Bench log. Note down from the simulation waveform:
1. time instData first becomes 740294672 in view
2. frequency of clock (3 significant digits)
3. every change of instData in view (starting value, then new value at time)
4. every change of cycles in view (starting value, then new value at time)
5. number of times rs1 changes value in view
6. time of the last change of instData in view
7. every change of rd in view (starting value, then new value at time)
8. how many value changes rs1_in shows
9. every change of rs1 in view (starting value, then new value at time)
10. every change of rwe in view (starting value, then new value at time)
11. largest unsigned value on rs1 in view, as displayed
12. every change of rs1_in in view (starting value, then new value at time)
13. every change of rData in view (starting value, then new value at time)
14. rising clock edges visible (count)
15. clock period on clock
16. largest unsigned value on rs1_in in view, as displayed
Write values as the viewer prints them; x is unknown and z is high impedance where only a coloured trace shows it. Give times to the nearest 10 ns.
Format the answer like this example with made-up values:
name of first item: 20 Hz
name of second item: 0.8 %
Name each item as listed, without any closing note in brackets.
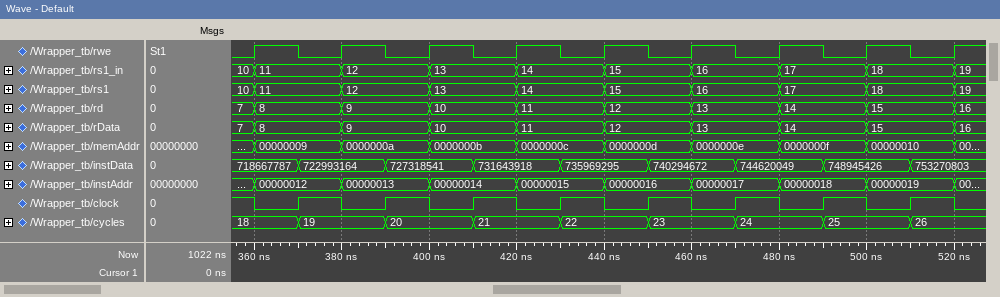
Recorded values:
time instData first becomes 740294672 in view: 450 ns
frequency of clock: 50.0 MHz
every change of instData in view: 718667787, 722993164 at 370 ns, 727318541 at 390 ns, 731643918 at 410 ns, 735969295 at 430 ns, 740294672 at 450 ns, 744620049 at 470 ns, 748945426 at 490 ns, 753270803 at 510 ns
every change of cycles in view: 18, 19 at 370 ns, 20 at 390 ns, 21 at 410 ns, 22 at 430 ns, 23 at 450 ns, 24 at 470 ns, 25 at 490 ns, 26 at 510 ns
number of times rs1 changes value in view: 9
time of the last change of instData in view: 510 ns
every change of rd in view: 7, 8 at 360 ns, 9 at 380 ns, 10 at 400 ns, 11 at 420 ns, 12 at 440 ns, 13 at 460 ns, 14 at 480 ns, 15 at 500 ns, 16 at 520 ns
how many value changes rs1_in shows: 9
every change of rs1 in view: 10, 11 at 360 ns, 12 at 380 ns, 13 at 400 ns, 14 at 420 ns, 15 at 440 ns, 16 at 460 ns, 17 at 480 ns, 18 at 500 ns, 19 at 520 ns
every change of rwe in view: 0, 1 at 360 ns, 0 at 370 ns, 1 at 380 ns, 0 at 390 ns, 1 at 400 ns, 0 at 410 ns, 1 at 420 ns, 0 at 430 ns, 1 at 440 ns, 0 at 450 ns, 1 at 460 ns, 0 at 470 ns, 1 at 480 ns, 0 at 490 ns, 1 at 500 ns, 0 at 510 ns, 1 at 520 ns
largest unsigned value on rs1 in view, as displayed: 19
every change of rs1_in in view: 10, 11 at 360 ns, 12 at 380 ns, 13 at 400 ns, 14 at 420 ns, 15 at 440 ns, 16 at 460 ns, 17 at 480 ns, 18 at 500 ns, 19 at 520 ns
every change of rData in view: 7, 8 at 360 ns, 9 at 380 ns, 10 at 400 ns, 11 at 420 ns, 12 at 440 ns, 13 at 460 ns, 14 at 480 ns, 15 at 500 ns, 16 at 520 ns
rising clock edges visible: 8
clock period on clock: 20 ns
largest unsigned value on rs1_in in view, as displayed: 19
